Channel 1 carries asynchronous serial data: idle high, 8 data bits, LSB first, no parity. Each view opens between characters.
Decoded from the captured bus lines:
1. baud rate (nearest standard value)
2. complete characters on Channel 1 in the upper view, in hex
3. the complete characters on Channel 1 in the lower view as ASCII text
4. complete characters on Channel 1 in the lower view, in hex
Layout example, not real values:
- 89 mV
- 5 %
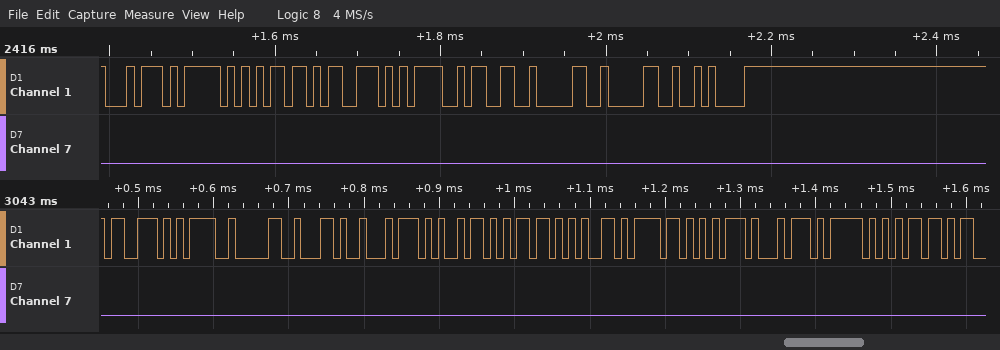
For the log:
- 115200 baud
- 74, 5F, 6D, 73, 3D, 33, 30, 30, 0A
- "s=0,timeout_m"
- 73, 3D, 30, 2C, 74, 69, 6D, 65, 6F, 75, 74, 5F, 6D
